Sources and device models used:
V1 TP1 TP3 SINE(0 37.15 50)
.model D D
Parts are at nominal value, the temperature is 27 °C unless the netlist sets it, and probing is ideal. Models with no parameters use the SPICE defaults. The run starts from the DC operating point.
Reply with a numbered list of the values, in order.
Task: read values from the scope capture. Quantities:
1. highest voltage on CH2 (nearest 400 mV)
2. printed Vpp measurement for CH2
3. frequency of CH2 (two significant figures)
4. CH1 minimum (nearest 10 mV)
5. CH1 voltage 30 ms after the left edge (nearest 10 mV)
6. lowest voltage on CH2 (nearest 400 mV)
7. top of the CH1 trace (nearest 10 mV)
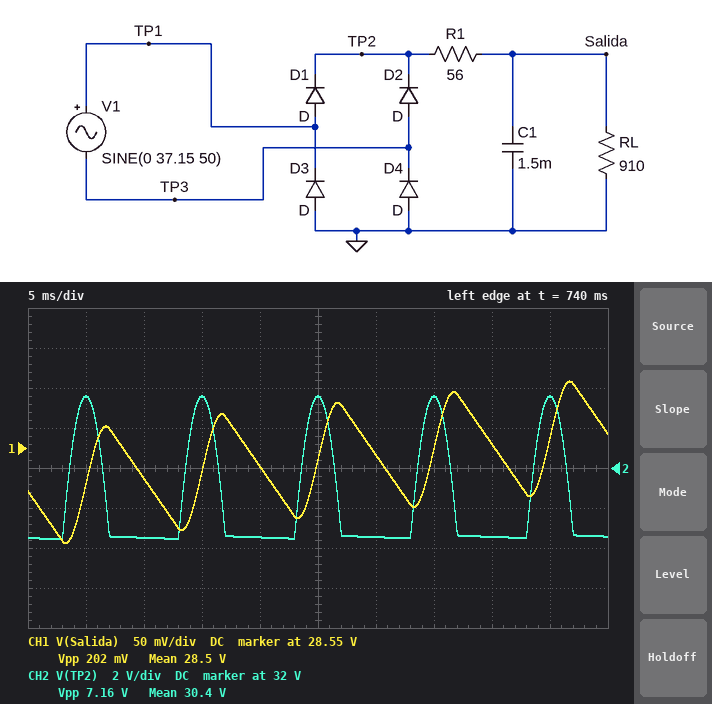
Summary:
1. 35.6 V
2. 7.16 V
3. 100 Hz
4. 28.43 V
5. 28.54 V
6. 28.4 V
7. 28.63 V
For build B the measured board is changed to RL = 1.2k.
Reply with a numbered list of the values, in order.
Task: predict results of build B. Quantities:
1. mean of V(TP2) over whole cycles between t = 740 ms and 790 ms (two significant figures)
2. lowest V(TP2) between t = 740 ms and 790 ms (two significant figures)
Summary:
1. 31 V
2. 29 V
